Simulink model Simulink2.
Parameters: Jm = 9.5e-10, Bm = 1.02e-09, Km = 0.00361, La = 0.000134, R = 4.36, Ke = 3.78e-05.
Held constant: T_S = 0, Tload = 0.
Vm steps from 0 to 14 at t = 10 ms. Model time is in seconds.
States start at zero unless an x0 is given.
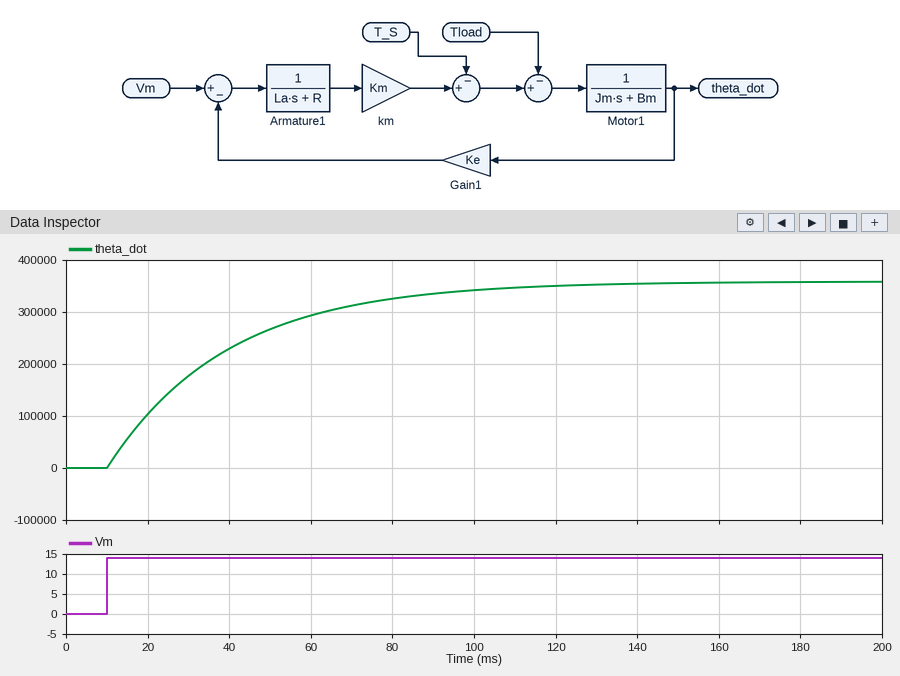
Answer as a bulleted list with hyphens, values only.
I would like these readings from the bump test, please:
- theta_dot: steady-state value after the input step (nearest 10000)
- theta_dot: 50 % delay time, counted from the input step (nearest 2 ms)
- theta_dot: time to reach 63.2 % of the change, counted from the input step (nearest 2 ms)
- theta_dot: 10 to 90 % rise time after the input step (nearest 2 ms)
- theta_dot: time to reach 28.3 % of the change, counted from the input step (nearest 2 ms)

- 360000
- 20 ms
- 30 ms
- 64 ms
- 10 ms
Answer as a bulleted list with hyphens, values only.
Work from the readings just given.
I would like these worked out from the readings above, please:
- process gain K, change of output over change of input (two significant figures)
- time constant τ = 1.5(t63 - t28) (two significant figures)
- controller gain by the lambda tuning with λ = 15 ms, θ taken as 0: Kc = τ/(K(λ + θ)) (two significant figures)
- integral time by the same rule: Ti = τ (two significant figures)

- 26000
- 30 ms
- 0.000077
- 30 ms
